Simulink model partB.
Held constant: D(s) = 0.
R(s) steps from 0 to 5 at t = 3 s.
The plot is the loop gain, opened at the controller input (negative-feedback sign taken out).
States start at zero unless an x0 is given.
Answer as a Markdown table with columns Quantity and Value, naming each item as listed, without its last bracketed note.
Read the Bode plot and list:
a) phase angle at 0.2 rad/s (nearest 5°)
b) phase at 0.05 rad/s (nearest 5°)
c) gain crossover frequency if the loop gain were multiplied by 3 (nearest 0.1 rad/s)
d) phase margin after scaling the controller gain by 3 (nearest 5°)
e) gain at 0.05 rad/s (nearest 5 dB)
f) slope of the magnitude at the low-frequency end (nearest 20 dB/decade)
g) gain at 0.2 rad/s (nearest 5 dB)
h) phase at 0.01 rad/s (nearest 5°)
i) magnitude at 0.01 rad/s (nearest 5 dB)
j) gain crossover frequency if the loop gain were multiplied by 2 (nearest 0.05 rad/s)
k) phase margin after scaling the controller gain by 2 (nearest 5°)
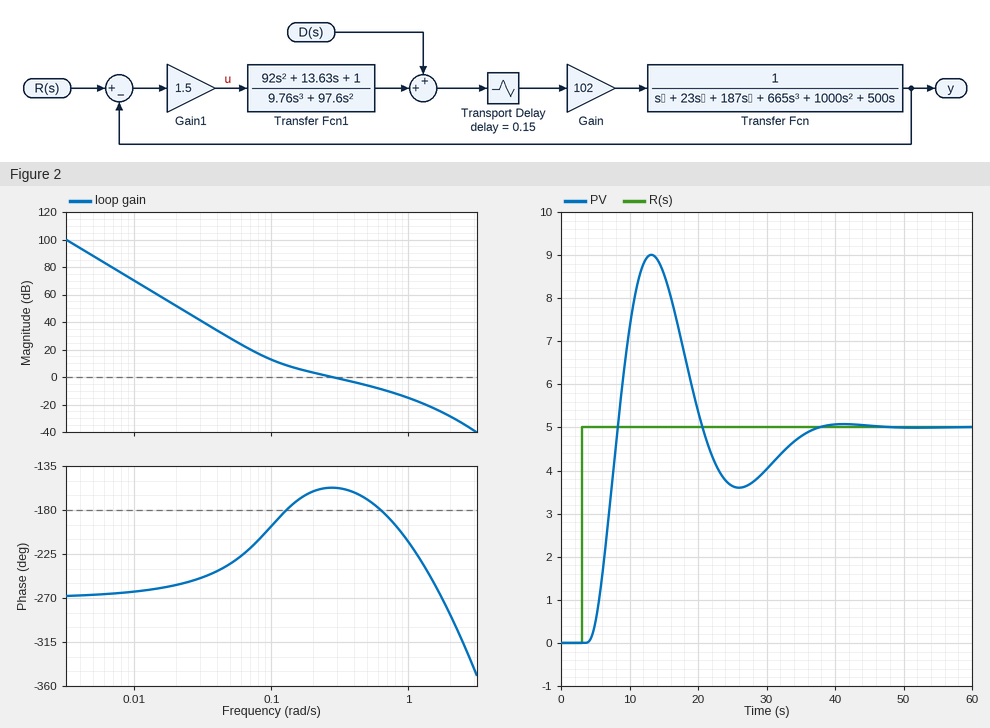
| Quantity | Value |
|---|---|
| phase angle at 0.2 rad/s | -160° |
| phase at 0.05 rad/s | -235° |
| gain crossover frequency if the loop gain were multiplied by 3 | 0.7 rad/s |
| phase margin after scaling the controller gain by 3 | -5° |
| gain at 0.05 rad/s | 30 dB |
| slope of the magnitude at the low-frequency end | -60 dB/decade |
| gain at 0.2 rad/s | 5 dB |
| phase at 0.01 rad/s | -265° |
| magnitude at 0.01 rad/s | 70 dB |
| gain crossover frequency if the loop gain were multiplied by 2 | 0.50 rad/s |
| phase margin after scaling the controller gain by 2 | 10° |
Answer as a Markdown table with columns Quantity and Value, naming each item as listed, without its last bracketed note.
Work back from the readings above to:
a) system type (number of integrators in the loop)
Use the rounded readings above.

| Quantity | Value |
|---|---|
| system type | 3 |
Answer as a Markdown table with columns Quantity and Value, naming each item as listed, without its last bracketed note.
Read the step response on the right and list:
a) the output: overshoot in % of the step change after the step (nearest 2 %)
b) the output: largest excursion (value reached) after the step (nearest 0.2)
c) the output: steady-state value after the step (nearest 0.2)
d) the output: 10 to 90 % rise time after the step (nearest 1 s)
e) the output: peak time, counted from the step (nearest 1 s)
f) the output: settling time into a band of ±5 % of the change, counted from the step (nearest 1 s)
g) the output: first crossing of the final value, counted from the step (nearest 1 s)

| Quantity | Value |
|---|---|
| the output: overshoot in % of the step change after the step | 80 % |
| the output: largest excursion (value reached) after the step | 9.0 |
| the output: steady-state value after the step | 5.0 |
| the output: 10 to 90 % rise time after the step | 3 s |
| the output: peak time, counted from the step | 10 s |
| the output: settling time into a band of ±5 % of the change, counted from the step | 32 s |
| the output: first crossing of the final value, counted from the step | 5 s |
